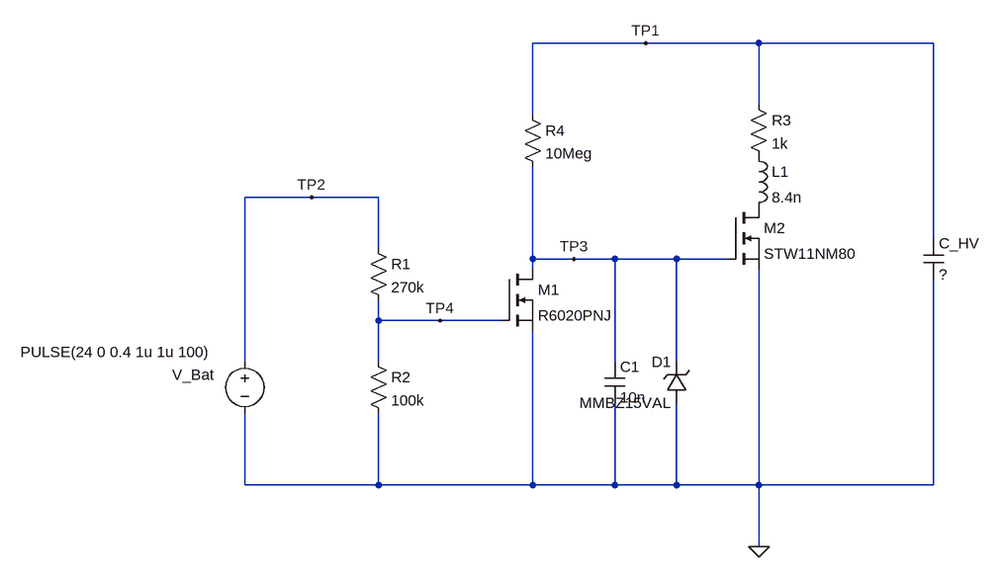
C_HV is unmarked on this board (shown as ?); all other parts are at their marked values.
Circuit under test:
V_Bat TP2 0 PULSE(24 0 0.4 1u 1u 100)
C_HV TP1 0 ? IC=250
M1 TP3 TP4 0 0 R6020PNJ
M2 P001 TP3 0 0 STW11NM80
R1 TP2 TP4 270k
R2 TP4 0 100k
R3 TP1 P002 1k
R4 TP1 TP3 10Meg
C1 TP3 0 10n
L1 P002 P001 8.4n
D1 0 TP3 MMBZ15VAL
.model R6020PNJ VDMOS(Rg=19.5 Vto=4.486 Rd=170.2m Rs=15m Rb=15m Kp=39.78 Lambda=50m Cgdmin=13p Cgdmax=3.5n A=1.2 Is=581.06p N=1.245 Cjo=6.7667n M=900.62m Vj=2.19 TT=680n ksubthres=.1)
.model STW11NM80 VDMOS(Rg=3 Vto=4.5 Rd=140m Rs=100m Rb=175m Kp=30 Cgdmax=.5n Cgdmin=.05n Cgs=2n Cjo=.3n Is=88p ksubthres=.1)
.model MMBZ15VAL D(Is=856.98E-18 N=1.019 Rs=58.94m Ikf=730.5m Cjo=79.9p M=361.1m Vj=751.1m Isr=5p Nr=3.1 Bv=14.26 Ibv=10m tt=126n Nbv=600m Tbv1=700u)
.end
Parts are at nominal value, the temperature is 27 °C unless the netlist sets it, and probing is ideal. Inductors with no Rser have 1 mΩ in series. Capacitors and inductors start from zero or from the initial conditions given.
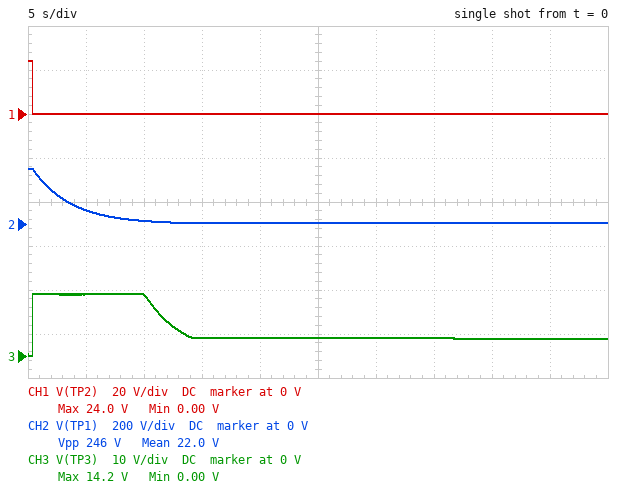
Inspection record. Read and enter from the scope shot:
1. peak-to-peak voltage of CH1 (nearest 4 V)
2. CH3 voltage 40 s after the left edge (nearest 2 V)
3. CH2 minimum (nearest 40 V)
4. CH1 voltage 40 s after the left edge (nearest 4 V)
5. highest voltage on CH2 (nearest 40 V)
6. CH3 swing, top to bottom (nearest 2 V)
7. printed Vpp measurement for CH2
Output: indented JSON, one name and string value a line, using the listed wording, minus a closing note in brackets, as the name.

{
  "peak-to-peak voltage of CH1": "24 V",
  "CH3 voltage 40 s after the left edge": "4 V",
  "CH2 minimum": "0 V",
  "CH1 voltage 40 s after the left edge": "0 V",
  "highest voltage on CH2": "240 V",
  "CH3 swing, top to bottom": "14 V",
  "printed Vpp measurement for CH2": "246 V"
}
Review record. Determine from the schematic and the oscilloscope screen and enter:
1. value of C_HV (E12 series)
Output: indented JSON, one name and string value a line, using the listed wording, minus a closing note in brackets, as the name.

{
  "value of C_HV": "3.3 mF"
}
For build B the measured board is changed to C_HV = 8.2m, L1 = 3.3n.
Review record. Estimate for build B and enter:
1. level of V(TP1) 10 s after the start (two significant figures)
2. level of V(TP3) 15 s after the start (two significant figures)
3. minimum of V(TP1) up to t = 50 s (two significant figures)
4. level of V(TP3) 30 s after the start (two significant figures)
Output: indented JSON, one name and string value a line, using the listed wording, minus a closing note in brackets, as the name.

{
  "level of V(TP1) 10 s after the start": "78 V",
  "level of V(TP3) 15 s after the start": "14 V",
  "minimum of V(TP1) up to t = 50 s": "4.1 V",
  "level of V(TP3) 30 s after the start": "6.9 V"
}
